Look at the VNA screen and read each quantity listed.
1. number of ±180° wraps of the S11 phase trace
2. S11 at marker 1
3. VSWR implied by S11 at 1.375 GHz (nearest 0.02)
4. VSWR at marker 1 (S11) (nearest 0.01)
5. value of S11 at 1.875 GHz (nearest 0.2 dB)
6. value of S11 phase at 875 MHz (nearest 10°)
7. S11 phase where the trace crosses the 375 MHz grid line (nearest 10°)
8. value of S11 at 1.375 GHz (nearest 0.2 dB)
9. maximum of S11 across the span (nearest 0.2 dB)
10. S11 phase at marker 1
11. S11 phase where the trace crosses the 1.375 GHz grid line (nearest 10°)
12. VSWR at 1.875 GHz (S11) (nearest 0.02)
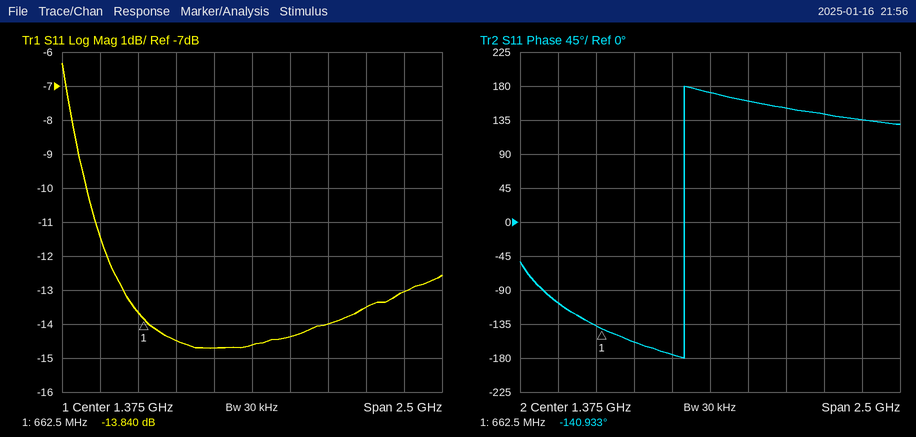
1
-13.840 dB
1.46
1.51
-14.0 dB
-160°
-110°
-14.6 dB
-6.4 dB
-140.933°
170°
1.50
